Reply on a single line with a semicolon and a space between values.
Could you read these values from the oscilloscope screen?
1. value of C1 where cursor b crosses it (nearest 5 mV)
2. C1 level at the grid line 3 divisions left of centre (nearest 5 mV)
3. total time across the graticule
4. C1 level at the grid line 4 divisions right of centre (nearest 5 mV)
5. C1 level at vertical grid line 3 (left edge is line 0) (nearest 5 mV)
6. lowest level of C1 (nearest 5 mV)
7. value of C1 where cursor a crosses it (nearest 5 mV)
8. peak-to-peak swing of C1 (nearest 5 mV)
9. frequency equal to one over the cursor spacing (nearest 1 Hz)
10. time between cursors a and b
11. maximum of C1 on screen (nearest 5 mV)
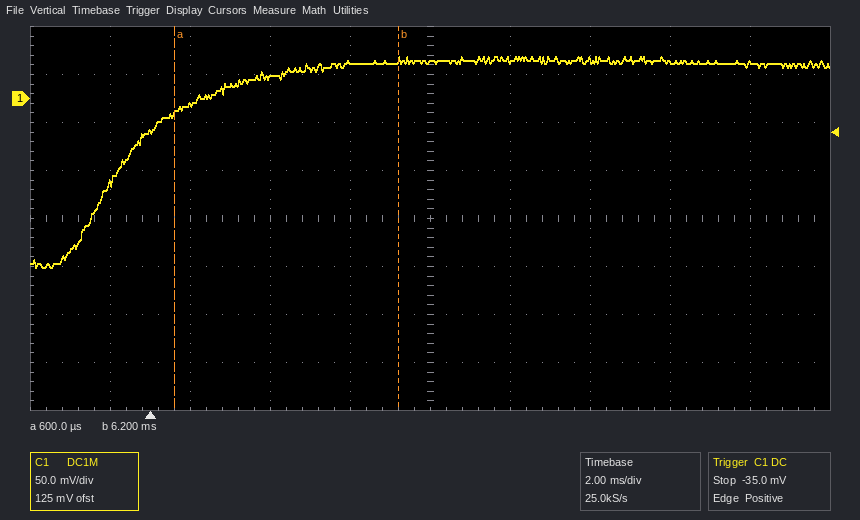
40 mV; -5 mV; 20 ms; 35 mV; 20 mV; -175 mV; -15 mV; 220 mV; 179 Hz; 5.6 ms; 45 mV
